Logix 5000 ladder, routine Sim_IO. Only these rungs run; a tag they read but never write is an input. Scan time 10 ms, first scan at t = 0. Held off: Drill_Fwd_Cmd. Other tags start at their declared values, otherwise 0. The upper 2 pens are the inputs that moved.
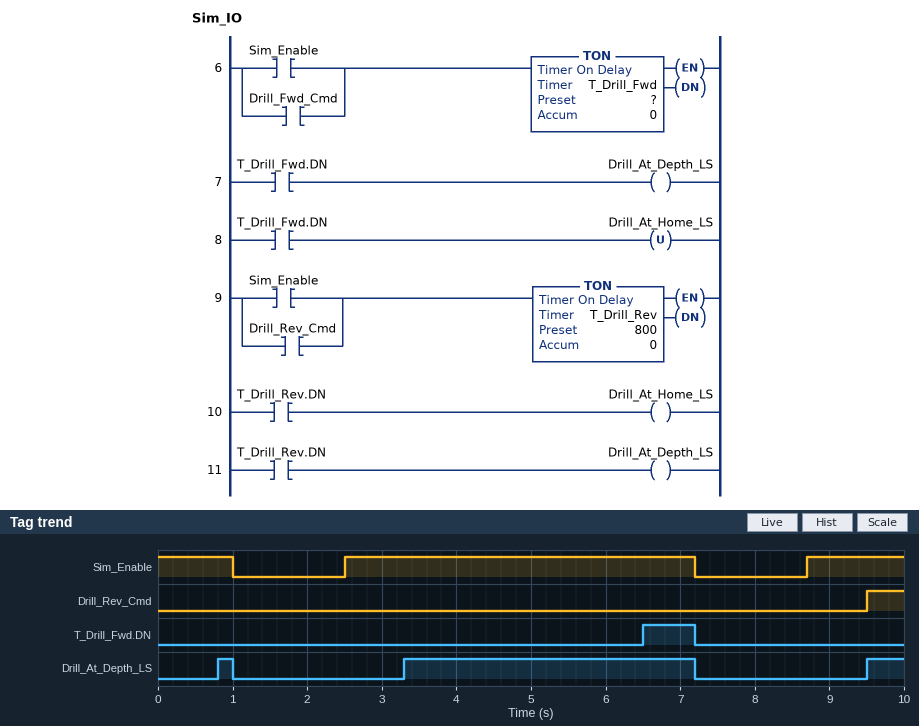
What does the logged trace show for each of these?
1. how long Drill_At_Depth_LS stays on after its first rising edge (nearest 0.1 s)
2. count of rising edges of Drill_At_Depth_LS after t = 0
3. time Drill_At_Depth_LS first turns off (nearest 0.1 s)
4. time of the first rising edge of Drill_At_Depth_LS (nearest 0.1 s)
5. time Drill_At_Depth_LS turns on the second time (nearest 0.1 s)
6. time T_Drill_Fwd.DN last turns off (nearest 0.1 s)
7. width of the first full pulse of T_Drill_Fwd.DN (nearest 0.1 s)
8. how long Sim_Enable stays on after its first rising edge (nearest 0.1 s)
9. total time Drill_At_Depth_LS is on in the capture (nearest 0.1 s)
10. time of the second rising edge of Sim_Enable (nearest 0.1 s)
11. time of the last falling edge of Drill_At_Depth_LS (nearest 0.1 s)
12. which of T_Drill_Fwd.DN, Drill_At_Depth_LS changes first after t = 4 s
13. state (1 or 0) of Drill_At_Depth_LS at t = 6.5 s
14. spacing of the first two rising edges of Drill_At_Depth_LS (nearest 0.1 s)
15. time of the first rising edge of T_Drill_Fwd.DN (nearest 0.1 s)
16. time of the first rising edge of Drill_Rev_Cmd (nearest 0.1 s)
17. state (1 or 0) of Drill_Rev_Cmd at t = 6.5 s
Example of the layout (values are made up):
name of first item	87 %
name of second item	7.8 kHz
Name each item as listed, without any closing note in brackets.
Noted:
how long Drill_At_Depth_LS stays on after its first rising edge	0.2 s
count of rising edges of Drill_At_Depth_LS after t = 0	3
time Drill_At_Depth_LS first turns off	1.0 s
time of the first rising edge of Drill_At_Depth_LS	0.8 s
time Drill_At_Depth_LS turns on the second time	3.3 s
time T_Drill_Fwd.DN last turns off	7.2 s
width of the first full pulse of T_Drill_Fwd.DN	0.7 s
how long Sim_Enable stays on after its first rising edge	4.7 s
total time Drill_At_Depth_LS is on in the capture	4.6 s
time of the second rising edge of Sim_Enable	8.7 s
time of the last falling edge of Drill_At_Depth_LS	7.2 s
which of T_Drill_Fwd.DN, Drill_At_Depth_LS changes first after t = 4 s	T_Drill_Fwd.DN
state (1 or 0) of Drill_At_Depth_LS at t = 6.5 s	1
spacing of the first two rising edges of Drill_At_Depth_LS	2.5 s
time of the first rising edge of T_Drill_Fwd.DN	6.5 s
time of the first rising edge of Drill_Rev_Cmd	9.5 s
state (1 or 0) of Drill_Rev_Cmd at t = 6.5 s	0
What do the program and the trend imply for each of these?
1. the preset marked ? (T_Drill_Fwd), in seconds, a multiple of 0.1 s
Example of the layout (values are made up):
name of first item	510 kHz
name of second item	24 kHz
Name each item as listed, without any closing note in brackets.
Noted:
the preset marked ? (T_Drill_Fwd), in seconds, a multiple of 0.1 s	4.0 s
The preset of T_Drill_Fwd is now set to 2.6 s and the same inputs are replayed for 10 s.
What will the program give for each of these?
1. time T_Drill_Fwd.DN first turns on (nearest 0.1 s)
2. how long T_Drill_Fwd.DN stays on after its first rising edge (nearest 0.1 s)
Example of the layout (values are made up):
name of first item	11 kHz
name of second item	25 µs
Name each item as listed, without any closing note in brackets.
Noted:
time T_Drill_Fwd.DN first turns on	5.1 s
how long T_Drill_Fwd.DN stays on after its first rising edge	2.1 s
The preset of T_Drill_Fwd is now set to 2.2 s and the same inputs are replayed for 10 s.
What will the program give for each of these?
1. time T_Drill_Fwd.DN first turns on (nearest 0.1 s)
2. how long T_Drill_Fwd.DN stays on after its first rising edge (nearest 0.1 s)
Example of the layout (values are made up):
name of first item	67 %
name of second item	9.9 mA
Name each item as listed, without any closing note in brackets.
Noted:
time T_Drill_Fwd.DN first turns on	4.7 s
how long T_Drill_Fwd.DN stays on after its first rising edge	2.5 s
